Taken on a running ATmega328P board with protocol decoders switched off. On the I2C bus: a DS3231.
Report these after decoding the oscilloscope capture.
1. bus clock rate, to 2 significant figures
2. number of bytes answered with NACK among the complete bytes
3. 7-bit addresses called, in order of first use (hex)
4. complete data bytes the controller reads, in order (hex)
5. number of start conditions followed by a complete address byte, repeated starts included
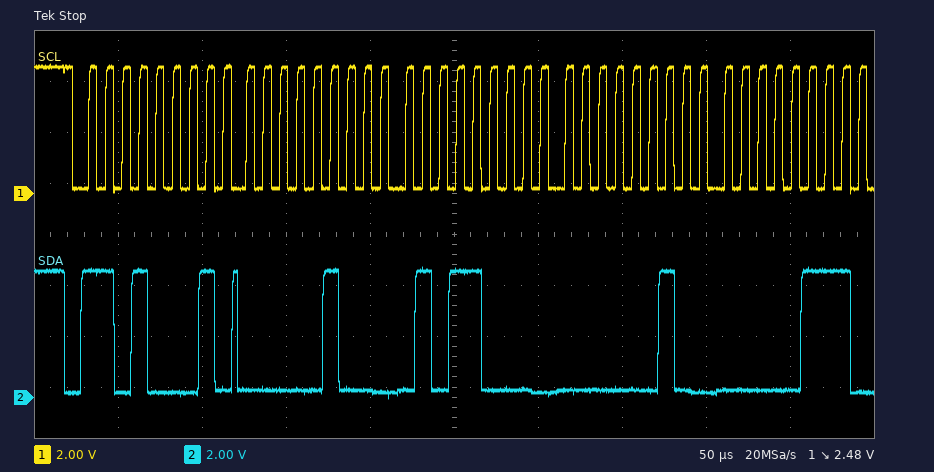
100 kHz
0
0x68
04 58 02 07
1
